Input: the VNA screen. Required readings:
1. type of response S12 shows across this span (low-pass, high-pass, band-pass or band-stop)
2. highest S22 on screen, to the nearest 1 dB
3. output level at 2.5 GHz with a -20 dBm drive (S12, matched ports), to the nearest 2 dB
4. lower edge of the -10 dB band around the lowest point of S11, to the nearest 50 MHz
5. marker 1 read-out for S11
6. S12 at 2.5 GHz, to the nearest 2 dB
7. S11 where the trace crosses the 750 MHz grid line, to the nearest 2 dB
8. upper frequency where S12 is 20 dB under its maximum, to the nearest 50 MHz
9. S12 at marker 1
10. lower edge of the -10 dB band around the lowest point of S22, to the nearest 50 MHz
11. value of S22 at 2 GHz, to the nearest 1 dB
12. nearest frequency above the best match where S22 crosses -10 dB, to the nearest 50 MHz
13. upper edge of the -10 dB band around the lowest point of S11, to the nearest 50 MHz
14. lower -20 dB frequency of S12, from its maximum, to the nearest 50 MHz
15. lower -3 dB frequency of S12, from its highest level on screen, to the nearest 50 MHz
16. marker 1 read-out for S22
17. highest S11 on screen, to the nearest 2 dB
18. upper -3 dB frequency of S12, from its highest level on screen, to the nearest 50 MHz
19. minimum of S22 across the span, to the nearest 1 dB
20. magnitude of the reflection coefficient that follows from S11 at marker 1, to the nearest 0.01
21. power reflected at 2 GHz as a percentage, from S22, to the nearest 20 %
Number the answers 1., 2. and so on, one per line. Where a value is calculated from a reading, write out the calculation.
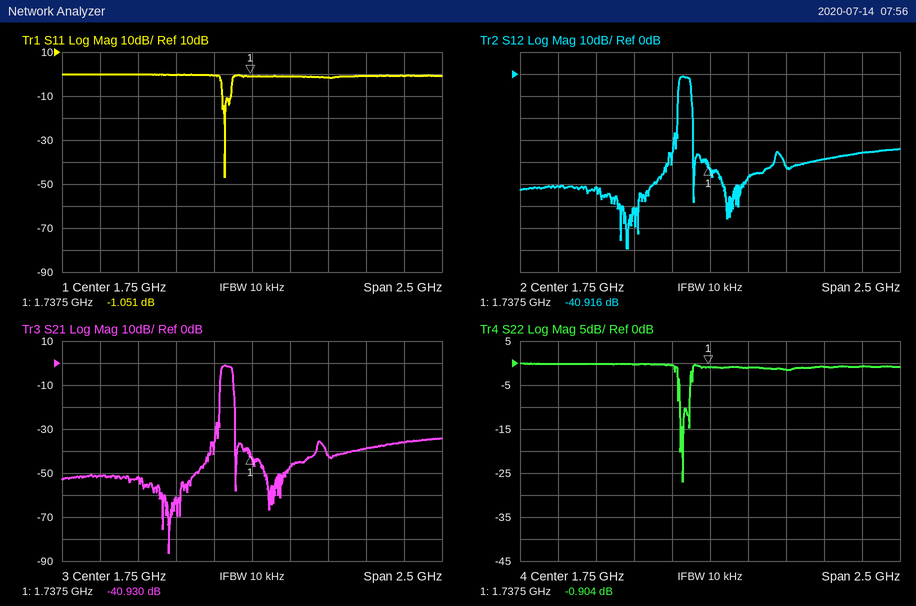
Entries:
1. band-pass
2. 0 dB
3. -20 dBm + (-38 dB) = -58 dBm
4. 1.55 GHz
5. -1.051 dB
6. -38 dB
7. 0 dB
8. 1.65 GHz
9. -40.916 dB
10. 1.55 GHz
11. -1 dB
12. 1.60 GHz
13. 1.60 GHz
14. 1.55 GHz
15. 1.55 GHz
16. -0.904 dB
17. 0 dB
18. 1.60 GHz
19. -27 dB
20. 10^(-1.051/20) ≈ 0.89
21. 10^(-1/10) ≈ 79.4 %, so 80 % to the nearest 20 %
